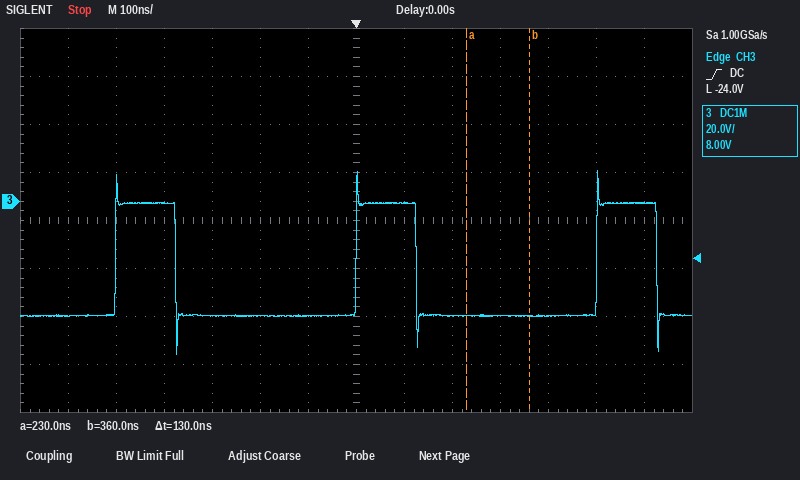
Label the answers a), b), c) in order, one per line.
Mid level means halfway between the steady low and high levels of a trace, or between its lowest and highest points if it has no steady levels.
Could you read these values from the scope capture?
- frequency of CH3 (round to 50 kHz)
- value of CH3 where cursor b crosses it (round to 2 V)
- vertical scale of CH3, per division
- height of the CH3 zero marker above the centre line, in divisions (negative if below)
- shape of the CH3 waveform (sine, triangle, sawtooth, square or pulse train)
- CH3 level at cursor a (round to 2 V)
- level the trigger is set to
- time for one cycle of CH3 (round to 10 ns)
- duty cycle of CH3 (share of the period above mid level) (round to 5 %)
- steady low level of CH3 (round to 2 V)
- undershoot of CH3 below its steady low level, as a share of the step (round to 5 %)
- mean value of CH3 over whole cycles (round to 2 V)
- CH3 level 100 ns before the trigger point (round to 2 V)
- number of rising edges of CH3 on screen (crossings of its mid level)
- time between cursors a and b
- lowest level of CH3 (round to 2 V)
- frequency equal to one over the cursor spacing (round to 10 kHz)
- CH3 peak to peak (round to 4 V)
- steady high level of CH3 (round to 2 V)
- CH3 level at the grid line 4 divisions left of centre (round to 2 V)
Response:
a) 2.00 MHz
b) -48 V
c) 20 V
d) +0.4 div
e) pulse train
f) -48 V
g) -24.0 V
h) 500 ns
i) 25 %
j) -48 V
k) 35 %
l) -36 V
m) -48 V
n) 3
o) 130 ns
p) -64 V
q) 7.69 MHz
r) 76 V
s) 0 V
t) 0 V
